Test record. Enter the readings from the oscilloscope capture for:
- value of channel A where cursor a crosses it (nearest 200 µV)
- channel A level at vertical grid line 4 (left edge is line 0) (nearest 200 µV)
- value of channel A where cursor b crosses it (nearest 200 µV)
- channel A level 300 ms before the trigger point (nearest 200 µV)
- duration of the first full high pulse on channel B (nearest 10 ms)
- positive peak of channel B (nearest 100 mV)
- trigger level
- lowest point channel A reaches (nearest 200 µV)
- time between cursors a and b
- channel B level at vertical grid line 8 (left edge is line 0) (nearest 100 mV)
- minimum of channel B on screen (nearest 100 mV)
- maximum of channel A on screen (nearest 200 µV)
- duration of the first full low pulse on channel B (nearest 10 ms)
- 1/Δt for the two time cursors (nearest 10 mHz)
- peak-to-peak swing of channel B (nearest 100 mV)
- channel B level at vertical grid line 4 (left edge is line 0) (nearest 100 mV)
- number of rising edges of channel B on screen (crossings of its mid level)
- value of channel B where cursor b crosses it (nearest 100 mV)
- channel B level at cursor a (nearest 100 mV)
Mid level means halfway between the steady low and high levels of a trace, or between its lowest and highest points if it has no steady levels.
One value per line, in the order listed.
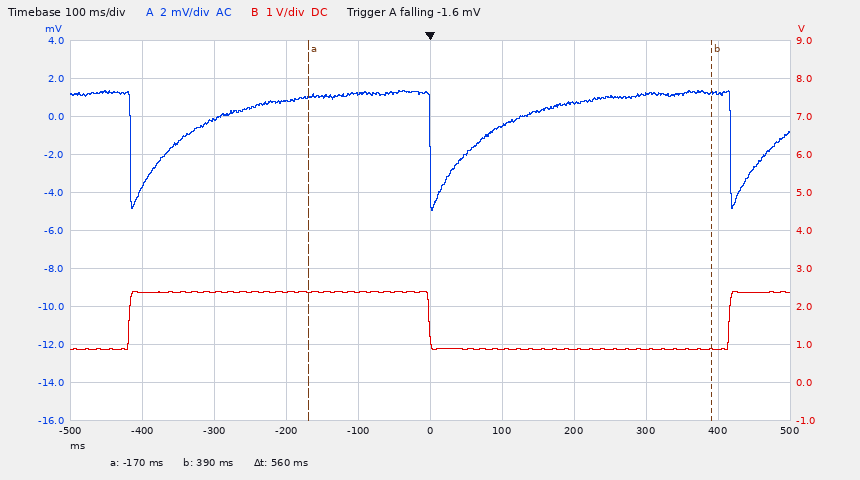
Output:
1.0 mV
1.2 mV
1.2 mV
-200 µV
420 ms
2.4 V
-1.6 mV
-5.0 mV
560 ms
900 mV
900 mV
1.4 mV
420 ms
1.79 Hz
1.5 V
2.4 V
2
900 mV
2.4 V
